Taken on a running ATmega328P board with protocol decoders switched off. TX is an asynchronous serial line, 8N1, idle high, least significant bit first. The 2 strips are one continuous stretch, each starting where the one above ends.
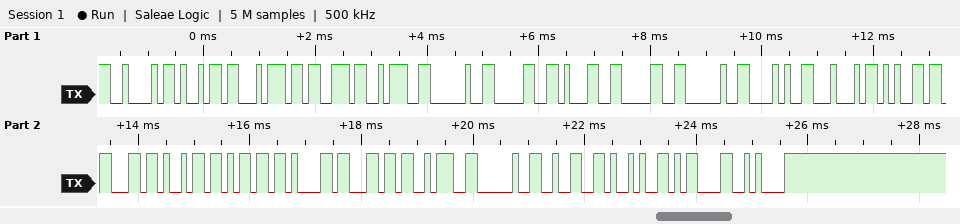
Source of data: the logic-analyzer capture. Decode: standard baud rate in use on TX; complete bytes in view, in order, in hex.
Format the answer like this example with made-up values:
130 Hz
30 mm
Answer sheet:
9600 baud
0x42 0x69 0x74 0x73 0x3A 0x20 0x30 0x31 0x30 0x20 0x28 0x44 0x65 0x63 0x69 0x6D 0x61 0x6C 0x3A 0x20 0x32 0x29 0x0D 0x0A
